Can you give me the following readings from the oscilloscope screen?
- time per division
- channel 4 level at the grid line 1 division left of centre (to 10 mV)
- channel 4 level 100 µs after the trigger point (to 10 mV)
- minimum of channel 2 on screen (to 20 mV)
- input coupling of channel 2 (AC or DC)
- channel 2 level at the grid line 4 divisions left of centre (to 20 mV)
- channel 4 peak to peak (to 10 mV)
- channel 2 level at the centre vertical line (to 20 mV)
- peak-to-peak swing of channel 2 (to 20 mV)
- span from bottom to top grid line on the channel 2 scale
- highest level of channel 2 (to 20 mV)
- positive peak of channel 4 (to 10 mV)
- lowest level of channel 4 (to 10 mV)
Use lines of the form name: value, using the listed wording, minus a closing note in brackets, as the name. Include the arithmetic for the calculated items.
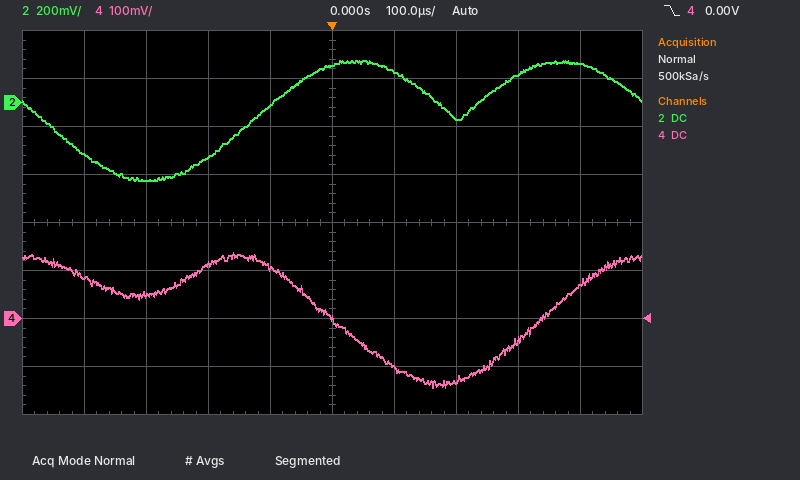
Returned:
time per division: 100 µs
channel 4 level at the grid line 1 division left of centre: 110 mV
channel 4 level 100 µs after the trigger point: -100 mV
minimum of channel 2 on screen: -320 mV
input coupling of channel 2: DC
channel 2 level at the grid line 4 divisions left of centre: -220 mV
channel 4 peak to peak: 140 mV − (-140 mV) = 280 mV
channel 2 level at the centre vertical line: 160 mV
peak-to-peak swing of channel 2: 180 mV − (-320 mV) = 500 mV
span from bottom to top grid line on the channel 2 scale: 1.6 V
highest level of channel 2: 180 mV
positive peak of channel 4: 140 mV
lowest level of channel 4: -140 mV
